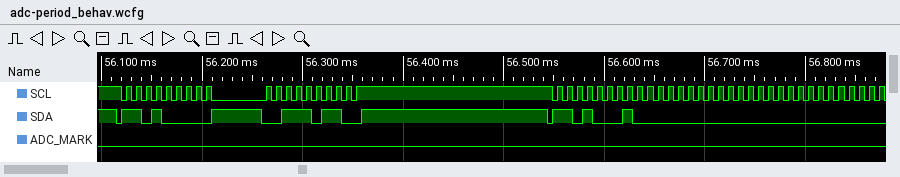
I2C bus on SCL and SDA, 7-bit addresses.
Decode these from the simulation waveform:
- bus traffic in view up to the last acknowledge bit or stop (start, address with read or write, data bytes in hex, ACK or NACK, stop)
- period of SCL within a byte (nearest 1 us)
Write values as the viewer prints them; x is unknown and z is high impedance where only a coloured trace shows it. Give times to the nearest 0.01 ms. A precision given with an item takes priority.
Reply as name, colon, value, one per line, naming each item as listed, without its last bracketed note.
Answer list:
bus traffic in view up to the last acknowledge bit or stop: start, address 68 write ACK, 3B ACK, stop, start, address 68 read ACK, 00 ACK, 00 ACK
period of SCL within a byte: 10 us
